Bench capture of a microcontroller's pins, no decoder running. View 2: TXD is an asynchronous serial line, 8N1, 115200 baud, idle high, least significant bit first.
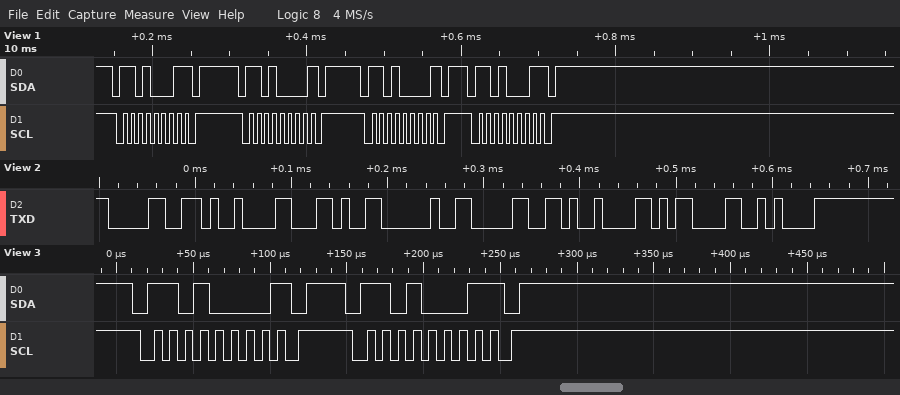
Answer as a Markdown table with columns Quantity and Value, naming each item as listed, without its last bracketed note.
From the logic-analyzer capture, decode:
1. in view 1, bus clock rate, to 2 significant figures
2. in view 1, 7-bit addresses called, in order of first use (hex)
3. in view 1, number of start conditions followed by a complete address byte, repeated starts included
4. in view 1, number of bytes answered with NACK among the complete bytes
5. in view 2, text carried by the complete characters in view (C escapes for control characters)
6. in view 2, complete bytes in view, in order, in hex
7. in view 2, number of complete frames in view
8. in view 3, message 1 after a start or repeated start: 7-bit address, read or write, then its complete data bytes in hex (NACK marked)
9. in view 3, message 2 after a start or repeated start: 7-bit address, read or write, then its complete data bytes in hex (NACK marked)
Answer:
| Quantity | Value |
|---|---|
| in view 1, bus clock rate, to 2 significant figures | 100 kHz |
| in view 1, 7-bit addresses called, in order of first use | 0x68 |
| in view 1, number of start conditions followed by a complete address byte, repeated starts included | 4 |
| in view 1, number of bytes answered with NACK among the complete bytes | 4 |
| in view 2, text carried by the complete characters in view | "0\t, 0\t\r\n" |
| in view 2, complete bytes in view, in order, in hex | 30 09 2C 20 30 09 0D 0A |
| in view 2, number of complete frames in view | 8 |
| in view 3, message 1 after a start or repeated start: 7-bit address, read or write, then its complete data bytes in hex | 0x68 write NACK |
| in view 3, message 2 after a start or repeated start: 7-bit address, read or write, then its complete data bytes in hex | 0x68 read NACK |
